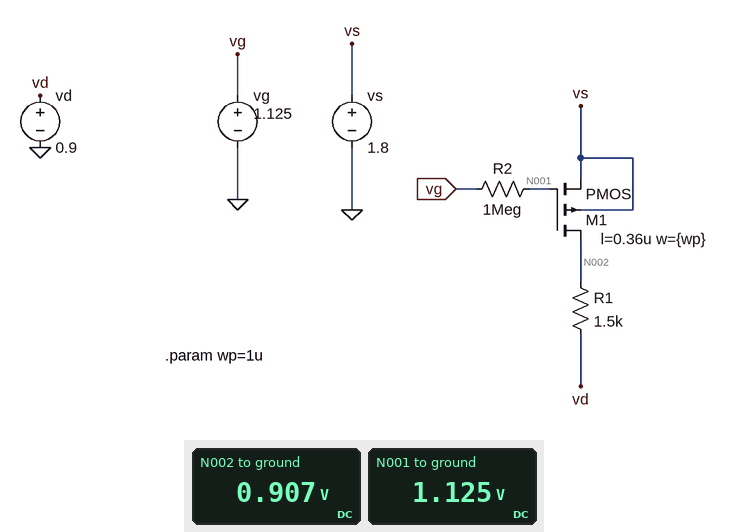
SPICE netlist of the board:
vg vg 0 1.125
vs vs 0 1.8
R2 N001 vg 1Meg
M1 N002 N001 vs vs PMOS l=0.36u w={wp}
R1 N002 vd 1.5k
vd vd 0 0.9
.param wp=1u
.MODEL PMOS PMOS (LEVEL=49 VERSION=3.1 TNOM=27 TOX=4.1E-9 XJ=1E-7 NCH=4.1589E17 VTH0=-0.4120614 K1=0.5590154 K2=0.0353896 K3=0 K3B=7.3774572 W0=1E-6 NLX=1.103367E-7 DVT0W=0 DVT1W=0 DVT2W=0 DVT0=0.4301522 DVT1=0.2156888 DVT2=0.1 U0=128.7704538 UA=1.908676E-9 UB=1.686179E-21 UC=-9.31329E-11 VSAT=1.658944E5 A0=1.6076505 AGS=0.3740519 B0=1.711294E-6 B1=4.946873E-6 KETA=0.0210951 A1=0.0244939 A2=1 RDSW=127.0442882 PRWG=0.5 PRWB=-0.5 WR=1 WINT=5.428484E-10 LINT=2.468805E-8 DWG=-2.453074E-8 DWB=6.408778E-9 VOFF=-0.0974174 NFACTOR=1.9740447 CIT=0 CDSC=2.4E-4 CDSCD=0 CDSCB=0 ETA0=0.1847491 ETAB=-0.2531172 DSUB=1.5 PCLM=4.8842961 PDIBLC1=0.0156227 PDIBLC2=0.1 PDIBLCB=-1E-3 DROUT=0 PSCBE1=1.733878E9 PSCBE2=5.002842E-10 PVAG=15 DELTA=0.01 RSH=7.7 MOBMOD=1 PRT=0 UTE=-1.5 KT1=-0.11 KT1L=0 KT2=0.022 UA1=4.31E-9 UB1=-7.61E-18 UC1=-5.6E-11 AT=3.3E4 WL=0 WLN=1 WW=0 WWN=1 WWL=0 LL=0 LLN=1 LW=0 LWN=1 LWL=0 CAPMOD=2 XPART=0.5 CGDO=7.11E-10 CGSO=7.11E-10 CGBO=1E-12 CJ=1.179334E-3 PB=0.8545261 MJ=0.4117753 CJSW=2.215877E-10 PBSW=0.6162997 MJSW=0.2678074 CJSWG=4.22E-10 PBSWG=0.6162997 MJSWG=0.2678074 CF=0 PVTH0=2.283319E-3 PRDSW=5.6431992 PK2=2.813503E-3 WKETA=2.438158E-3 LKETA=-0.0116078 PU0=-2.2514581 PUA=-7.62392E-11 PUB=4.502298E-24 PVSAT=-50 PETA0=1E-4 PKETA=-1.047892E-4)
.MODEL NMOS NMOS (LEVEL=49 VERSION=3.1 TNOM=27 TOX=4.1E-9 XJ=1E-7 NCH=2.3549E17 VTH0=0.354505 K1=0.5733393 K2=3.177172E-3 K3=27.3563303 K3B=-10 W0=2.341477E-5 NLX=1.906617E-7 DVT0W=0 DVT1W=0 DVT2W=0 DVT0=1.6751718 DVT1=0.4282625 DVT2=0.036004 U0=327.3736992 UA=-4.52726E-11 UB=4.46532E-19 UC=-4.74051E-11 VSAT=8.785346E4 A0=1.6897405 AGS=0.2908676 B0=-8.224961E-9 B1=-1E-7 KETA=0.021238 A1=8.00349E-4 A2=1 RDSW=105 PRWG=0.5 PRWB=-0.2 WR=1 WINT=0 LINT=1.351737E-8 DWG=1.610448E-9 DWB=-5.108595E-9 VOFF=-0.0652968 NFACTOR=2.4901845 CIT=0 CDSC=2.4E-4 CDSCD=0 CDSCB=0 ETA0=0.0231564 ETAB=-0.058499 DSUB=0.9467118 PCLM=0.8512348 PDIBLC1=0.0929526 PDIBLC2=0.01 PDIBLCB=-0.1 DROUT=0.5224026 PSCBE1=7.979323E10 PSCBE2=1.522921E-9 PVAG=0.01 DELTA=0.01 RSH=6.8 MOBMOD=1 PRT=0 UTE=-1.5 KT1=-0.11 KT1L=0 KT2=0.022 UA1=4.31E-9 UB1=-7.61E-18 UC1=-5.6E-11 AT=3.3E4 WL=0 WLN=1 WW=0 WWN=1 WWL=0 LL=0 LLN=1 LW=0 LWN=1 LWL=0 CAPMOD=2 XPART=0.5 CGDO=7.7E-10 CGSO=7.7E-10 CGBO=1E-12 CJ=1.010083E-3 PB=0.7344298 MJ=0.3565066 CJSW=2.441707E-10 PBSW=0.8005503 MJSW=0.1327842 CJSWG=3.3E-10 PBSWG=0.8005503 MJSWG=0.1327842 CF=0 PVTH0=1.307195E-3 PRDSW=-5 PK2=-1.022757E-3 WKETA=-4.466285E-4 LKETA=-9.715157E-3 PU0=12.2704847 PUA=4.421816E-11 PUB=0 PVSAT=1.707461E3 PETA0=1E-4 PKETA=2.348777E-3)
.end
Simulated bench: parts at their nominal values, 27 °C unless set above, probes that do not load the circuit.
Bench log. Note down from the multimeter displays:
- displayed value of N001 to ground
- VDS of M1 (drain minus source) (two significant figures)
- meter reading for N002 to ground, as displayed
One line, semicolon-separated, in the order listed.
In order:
1.125 V; -890 mV; 0.907 V
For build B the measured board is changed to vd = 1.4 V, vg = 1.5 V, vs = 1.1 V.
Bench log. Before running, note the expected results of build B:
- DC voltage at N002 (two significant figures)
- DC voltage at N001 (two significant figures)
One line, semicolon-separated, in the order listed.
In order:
1.4 V; 1.5 V
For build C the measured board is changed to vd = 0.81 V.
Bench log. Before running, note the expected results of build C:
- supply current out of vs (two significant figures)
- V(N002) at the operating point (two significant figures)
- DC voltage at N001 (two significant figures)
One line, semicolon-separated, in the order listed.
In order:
4.4 µA; 820 mV; 1.1 V
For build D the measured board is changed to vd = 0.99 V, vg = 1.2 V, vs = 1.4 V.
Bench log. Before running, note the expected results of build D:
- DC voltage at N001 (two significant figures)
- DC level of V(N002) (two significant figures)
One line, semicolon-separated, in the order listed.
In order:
1.2 V; 990 mV
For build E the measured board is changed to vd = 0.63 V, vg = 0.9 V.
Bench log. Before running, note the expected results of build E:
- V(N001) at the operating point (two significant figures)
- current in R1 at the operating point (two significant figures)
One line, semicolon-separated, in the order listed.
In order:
900 mV; 17 µA
